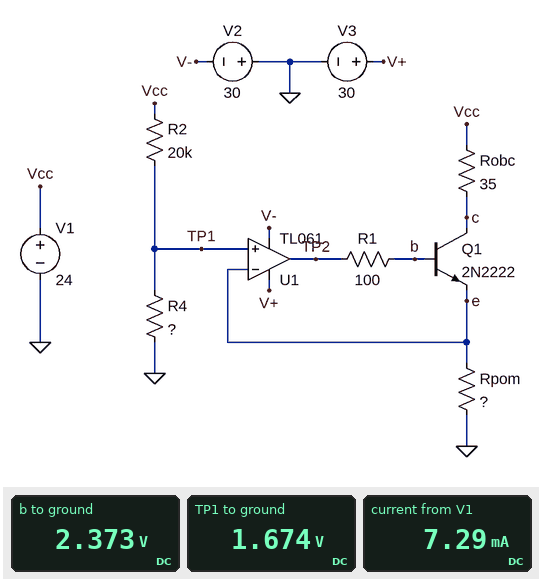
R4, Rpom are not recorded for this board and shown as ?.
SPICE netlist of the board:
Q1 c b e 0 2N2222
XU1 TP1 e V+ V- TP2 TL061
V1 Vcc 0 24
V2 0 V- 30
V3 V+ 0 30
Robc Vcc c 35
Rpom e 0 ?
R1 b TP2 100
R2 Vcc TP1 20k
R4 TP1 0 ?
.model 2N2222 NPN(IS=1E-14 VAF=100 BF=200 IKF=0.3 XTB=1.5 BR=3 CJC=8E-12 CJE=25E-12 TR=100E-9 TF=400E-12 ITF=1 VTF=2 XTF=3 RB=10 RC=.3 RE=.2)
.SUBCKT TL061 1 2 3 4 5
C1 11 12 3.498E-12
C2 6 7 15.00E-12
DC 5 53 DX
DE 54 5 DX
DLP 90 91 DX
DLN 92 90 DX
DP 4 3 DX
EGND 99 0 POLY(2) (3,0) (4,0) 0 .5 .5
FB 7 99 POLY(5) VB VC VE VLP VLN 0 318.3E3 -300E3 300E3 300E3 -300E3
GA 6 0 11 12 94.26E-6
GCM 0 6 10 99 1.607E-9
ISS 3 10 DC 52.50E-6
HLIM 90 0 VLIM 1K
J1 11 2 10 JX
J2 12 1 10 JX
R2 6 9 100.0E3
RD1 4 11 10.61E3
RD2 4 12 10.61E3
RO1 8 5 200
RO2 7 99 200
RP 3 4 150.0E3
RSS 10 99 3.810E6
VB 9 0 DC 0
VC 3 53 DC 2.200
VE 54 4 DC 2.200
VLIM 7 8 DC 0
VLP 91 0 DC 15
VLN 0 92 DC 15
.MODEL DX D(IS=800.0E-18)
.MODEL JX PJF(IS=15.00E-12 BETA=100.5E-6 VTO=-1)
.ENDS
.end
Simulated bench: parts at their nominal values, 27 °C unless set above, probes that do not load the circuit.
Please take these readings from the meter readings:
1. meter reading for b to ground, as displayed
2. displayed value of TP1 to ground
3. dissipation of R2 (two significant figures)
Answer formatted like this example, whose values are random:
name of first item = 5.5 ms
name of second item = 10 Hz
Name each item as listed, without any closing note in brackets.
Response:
meter reading for b to ground, as displayed = 2.373 V
displayed value of TP1 to ground = 1.674 V
dissipation of R2 = 25 mW
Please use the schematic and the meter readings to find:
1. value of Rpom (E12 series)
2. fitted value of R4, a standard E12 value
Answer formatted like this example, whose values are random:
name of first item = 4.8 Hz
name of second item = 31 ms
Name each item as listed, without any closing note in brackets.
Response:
value of Rpom = 270 Ω
fitted value of R4, a standard E12 value = 1.5 kΩ
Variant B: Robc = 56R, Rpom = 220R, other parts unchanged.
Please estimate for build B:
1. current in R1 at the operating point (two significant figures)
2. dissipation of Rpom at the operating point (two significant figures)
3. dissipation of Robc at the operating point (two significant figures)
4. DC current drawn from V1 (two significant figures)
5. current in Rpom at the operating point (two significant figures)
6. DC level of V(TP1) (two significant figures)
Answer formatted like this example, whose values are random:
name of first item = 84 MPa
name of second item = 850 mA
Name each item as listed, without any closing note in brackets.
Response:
current in R1 at the operating point = 32 µA
dissipation of Rpom at the operating point = 13 mW
dissipation of Robc at the operating point = 3.2 mW
DC current drawn from V1 = 8.7 mA
current in Rpom at the operating point = 7.6 mA
DC level of V(TP1) = 1.7 V
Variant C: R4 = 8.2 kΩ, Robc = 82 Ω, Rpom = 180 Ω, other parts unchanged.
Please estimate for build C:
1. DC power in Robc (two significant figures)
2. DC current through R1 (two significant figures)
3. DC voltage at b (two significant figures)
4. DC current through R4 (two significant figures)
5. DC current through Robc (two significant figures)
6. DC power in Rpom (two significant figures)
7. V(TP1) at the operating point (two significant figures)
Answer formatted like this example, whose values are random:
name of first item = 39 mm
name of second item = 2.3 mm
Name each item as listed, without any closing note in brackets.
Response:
DC power in Robc = 120 mW
DC current through R1 = 190 µA
DC voltage at b = 7.7 V
DC current through R4 = 850 µA
DC current through Robc = 39 mA
DC power in Rpom = 270 mW
V(TP1) at the operating point = 7.0 V
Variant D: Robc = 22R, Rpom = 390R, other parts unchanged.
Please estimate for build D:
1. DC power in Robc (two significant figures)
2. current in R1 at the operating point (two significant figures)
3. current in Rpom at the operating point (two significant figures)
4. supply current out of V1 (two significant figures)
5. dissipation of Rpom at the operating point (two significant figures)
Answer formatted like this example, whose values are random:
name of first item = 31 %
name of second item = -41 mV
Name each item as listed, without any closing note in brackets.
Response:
DC power in Robc = 400 µW
current in R1 at the operating point = 18 µA
current in Rpom at the operating point = 4.3 mA
supply current out of V1 = 5.4 mA
dissipation of Rpom at the operating point = 7.2 mW
